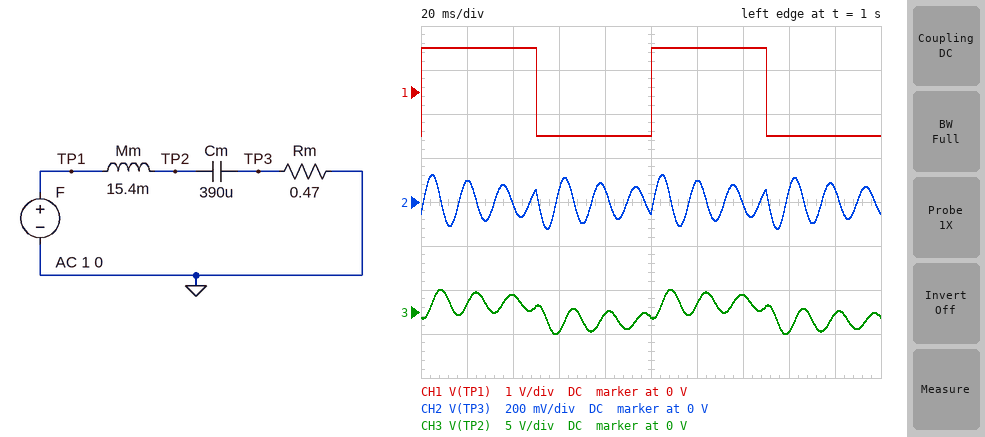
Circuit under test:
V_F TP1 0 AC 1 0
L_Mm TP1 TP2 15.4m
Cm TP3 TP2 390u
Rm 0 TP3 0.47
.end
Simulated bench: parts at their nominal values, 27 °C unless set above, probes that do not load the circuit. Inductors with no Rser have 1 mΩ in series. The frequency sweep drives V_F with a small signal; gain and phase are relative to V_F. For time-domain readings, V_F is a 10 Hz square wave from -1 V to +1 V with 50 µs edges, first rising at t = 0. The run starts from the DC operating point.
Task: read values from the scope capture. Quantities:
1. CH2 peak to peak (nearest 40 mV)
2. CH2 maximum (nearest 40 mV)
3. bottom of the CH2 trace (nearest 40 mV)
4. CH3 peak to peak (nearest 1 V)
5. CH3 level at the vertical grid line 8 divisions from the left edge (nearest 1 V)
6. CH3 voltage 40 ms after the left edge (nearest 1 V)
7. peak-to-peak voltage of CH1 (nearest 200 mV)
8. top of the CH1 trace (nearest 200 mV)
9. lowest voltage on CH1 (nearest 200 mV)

240 mV
120 mV
-120 mV
5 V
-2 V
2 V
2.0 V
1.0 V
-1.0 V
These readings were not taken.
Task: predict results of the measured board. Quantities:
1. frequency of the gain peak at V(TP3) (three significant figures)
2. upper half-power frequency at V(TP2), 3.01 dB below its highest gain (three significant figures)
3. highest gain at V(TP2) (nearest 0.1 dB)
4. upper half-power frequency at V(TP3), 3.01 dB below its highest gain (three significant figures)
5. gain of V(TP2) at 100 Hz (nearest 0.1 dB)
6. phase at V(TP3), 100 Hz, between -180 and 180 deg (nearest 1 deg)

64.9 Hz
67.2 Hz
22.5 dB
67.4 Hz
-2.7 dB
-85 deg
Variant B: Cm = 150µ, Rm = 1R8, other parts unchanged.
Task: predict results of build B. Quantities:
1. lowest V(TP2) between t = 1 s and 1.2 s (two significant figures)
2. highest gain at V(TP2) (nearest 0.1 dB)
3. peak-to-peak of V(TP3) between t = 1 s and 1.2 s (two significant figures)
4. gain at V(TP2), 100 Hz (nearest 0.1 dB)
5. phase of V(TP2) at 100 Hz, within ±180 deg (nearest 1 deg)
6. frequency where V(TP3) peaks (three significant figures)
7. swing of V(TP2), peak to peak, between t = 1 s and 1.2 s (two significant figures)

-2.5 V
15.2 dB
610 mV
14.5 dB
-53 deg
105 Hz
5.0 V
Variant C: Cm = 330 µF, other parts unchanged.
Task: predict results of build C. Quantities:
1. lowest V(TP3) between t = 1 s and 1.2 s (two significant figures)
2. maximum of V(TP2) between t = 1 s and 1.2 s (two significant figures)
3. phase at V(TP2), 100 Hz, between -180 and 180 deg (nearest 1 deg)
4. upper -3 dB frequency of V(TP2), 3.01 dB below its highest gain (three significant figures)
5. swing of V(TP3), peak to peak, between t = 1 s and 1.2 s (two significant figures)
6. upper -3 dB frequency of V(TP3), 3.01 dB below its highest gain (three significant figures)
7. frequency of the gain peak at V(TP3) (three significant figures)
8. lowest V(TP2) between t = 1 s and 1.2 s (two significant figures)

-240 mV
4.3 V
-169 deg
72.9 Hz
480 mV
73.1 Hz
70.6 Hz
-4.3 V
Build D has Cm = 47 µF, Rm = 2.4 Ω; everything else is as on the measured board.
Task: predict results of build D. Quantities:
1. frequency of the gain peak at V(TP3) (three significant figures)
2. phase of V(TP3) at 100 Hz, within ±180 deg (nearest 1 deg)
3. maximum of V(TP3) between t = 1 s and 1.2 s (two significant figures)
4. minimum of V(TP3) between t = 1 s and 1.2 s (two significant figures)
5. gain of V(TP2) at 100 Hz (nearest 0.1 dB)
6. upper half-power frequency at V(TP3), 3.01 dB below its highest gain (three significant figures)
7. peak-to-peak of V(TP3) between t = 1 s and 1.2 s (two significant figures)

187 Hz
84 deg
240 mV
-240 mV
2.9 dB
200 Hz
480 mV
